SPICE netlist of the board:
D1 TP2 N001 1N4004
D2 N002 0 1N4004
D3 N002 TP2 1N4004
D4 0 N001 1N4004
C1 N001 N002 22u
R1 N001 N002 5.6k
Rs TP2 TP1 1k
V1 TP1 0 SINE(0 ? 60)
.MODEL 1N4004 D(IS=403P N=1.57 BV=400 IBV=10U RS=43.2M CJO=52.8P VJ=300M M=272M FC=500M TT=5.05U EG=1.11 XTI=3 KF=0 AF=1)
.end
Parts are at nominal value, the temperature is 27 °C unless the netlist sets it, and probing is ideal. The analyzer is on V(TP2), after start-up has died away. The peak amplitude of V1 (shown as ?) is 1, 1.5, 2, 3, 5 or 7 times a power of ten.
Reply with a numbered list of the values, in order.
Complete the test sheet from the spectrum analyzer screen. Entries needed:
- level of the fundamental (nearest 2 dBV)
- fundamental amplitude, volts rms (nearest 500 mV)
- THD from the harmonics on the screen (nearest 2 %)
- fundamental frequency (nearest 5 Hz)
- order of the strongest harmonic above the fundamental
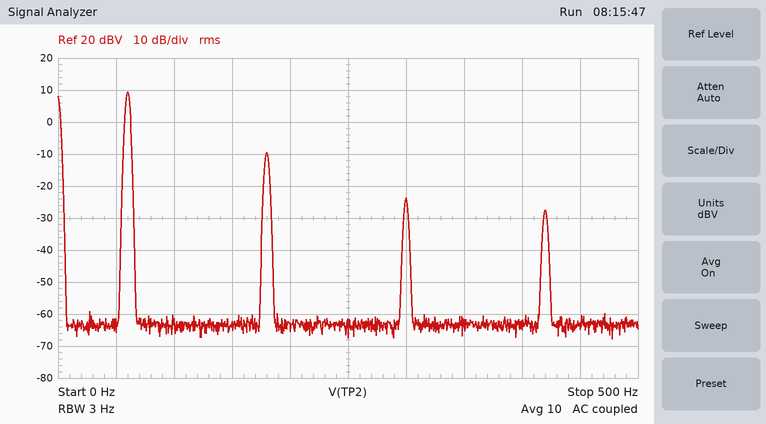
1. 10 dBV
2. 3.0 V
3. 12 %
4. 60 Hz
5. 3
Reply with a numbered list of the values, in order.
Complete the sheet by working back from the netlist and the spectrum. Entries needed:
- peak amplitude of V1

1. 5 V
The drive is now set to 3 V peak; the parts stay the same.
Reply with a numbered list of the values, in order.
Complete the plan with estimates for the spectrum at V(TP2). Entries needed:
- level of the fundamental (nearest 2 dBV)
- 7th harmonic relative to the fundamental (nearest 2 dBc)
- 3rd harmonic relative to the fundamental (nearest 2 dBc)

1. 6 dBV
2. -42 dBc
3. -20 dBc
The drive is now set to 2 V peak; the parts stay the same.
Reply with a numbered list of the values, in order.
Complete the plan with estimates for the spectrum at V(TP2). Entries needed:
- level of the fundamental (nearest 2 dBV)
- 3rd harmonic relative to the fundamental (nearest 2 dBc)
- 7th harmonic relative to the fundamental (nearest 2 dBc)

1. 2 dBV
2. -24 dBc
3. -52 dBc
